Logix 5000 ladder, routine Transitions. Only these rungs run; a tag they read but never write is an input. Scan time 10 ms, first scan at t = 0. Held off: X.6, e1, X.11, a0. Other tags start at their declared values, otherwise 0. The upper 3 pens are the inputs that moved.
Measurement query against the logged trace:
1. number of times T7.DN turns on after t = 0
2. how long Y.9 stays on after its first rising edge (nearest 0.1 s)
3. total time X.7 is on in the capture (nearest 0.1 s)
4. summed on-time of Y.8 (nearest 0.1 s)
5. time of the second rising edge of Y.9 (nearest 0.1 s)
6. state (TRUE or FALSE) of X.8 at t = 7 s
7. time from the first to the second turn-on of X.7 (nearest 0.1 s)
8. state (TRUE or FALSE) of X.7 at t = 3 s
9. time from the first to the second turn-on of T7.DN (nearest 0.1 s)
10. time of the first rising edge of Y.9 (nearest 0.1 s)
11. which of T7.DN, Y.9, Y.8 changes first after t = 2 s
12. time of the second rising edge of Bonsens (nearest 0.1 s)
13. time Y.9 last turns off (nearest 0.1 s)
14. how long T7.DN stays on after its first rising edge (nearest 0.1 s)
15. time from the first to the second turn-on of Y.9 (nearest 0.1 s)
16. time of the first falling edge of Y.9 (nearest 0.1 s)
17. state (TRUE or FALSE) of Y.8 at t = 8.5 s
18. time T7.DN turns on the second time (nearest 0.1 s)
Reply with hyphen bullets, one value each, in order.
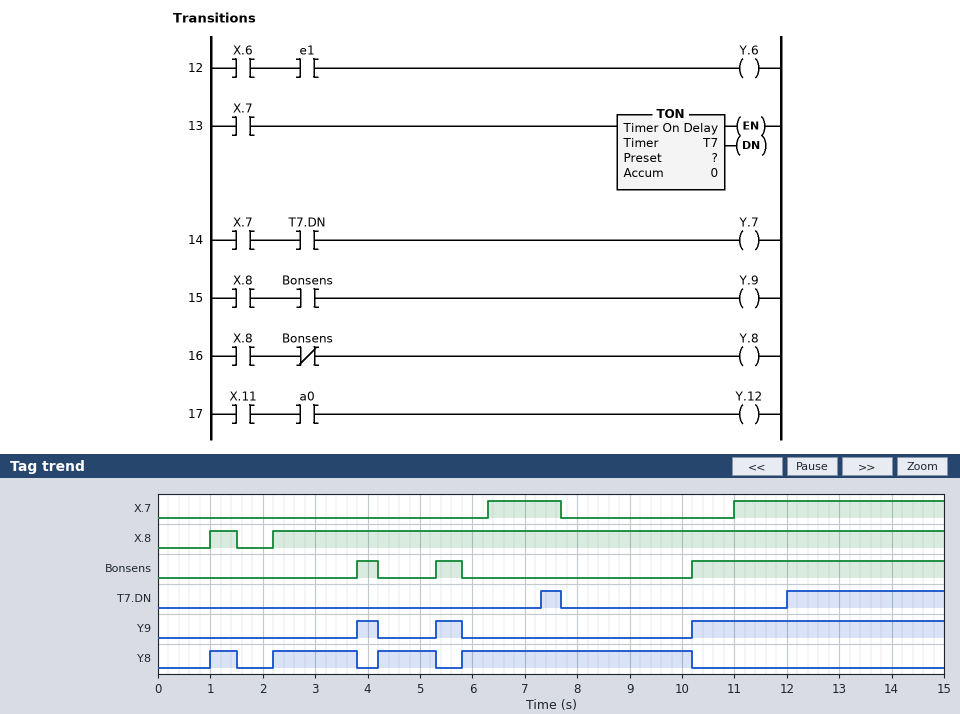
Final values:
- 2
- 0.4 s
- 5.4 s
- 7.6 s
- 5.3 s
- TRUE
- 4.7 s
- FALSE
- 4.7 s
- 3.8 s
- Y.8
- 5.3 s
- 5.8 s
- 0.4 s
- 1.5 s
- 4.2 s
- TRUE
- 12.0 s
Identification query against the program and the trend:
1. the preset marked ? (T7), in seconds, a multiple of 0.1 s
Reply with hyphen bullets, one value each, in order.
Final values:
- 1.0 s
